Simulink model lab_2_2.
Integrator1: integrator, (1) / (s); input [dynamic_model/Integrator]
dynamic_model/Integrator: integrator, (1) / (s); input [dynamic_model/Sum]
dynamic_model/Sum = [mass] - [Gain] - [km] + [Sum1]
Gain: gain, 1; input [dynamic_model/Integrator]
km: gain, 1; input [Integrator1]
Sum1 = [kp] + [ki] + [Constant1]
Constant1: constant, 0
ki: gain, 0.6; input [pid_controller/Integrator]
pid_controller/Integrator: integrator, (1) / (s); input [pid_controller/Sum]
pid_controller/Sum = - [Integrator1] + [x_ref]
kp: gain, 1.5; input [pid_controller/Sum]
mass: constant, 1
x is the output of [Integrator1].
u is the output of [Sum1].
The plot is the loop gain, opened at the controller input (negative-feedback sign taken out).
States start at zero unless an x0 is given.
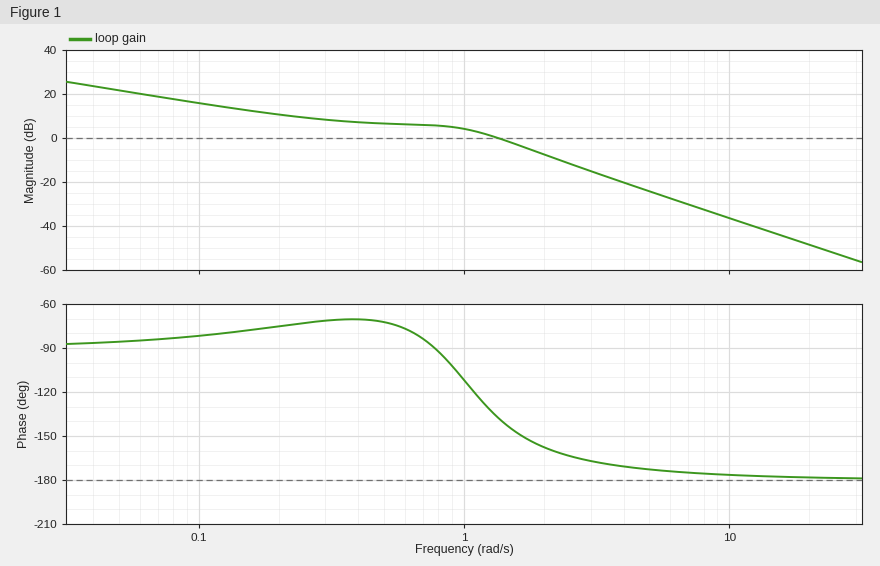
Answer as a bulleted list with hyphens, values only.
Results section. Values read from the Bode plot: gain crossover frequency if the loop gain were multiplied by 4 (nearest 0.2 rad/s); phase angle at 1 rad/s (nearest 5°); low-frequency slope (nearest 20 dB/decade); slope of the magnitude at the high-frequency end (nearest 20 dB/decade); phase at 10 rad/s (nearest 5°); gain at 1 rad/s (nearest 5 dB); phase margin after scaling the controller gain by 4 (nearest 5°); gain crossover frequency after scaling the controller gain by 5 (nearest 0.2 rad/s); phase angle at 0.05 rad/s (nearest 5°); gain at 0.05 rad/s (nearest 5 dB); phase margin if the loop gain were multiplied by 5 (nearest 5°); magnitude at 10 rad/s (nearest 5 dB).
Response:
- 2.6 rad/s
- -110°
- -20 dB/decade
- -40 dB/decade
- -175°
- 5 dB
- 15°
- 2.8 rad/s
- -85°
- 20 dB
- 15°
- -35 dB
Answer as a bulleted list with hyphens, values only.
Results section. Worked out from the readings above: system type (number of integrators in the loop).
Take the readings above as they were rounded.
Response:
- 1
